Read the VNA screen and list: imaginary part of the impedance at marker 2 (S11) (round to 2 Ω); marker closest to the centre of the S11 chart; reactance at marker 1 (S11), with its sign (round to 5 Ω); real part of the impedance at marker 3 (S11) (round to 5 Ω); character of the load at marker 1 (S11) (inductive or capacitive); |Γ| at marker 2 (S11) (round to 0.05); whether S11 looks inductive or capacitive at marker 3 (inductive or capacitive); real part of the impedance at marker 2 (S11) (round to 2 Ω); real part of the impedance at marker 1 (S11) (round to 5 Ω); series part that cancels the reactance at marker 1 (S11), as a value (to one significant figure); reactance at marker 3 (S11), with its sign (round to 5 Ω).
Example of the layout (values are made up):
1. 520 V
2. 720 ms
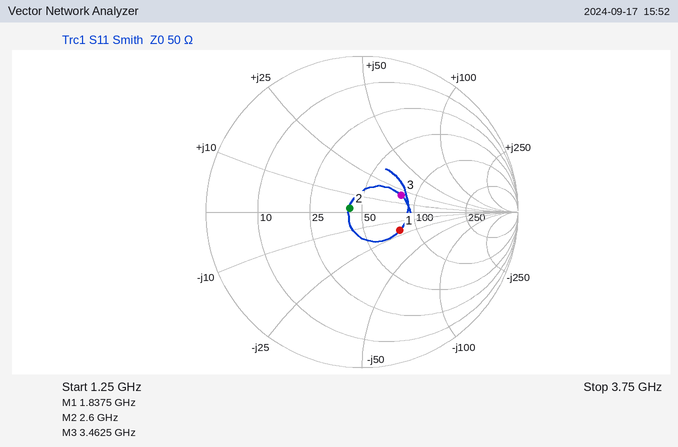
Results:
1. +2 Ω
2. marker 2
3. -20 Ω
4. 80 Ω
5. capacitive
6. 0.10
7. inductive
8. 42 Ω
9. 80 Ω
10. 2 nH
11. +20 Ω
